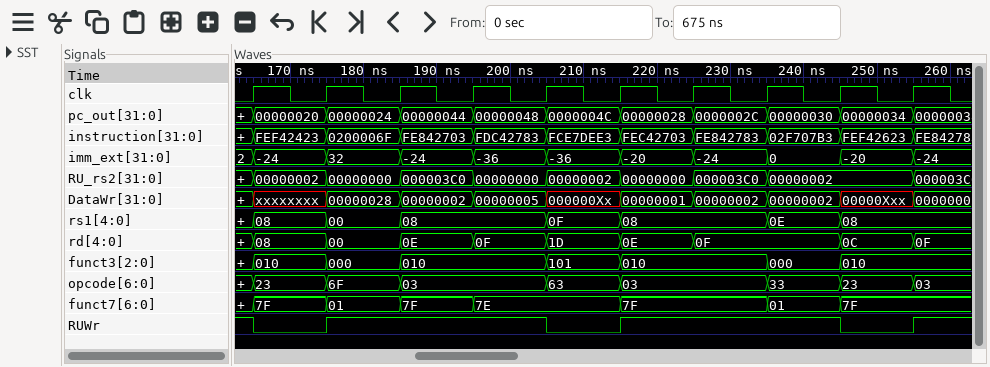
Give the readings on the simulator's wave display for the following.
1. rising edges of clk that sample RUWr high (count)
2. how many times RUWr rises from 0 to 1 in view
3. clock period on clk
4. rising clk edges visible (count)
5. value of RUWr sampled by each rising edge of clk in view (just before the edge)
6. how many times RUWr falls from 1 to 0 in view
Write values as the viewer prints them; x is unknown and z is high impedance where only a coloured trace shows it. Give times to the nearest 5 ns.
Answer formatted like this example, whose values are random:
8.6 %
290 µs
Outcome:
7
3
10 ns
10
1 0 1 1 1 0 1 1 1 0
3
